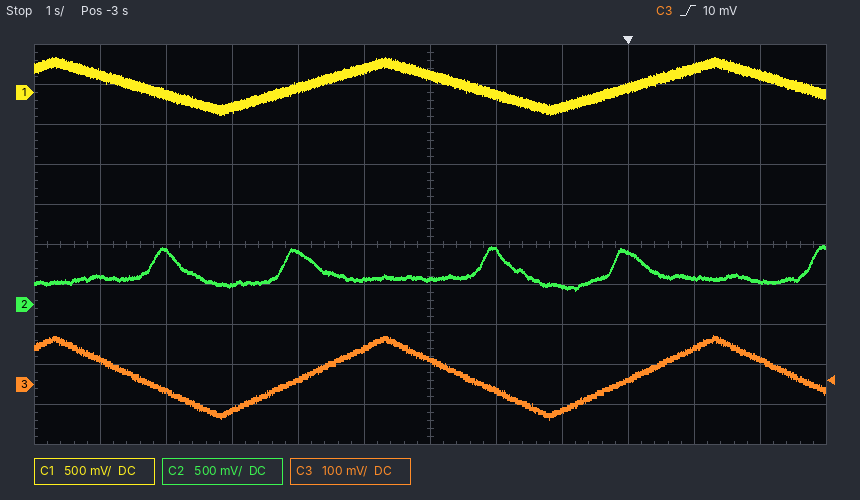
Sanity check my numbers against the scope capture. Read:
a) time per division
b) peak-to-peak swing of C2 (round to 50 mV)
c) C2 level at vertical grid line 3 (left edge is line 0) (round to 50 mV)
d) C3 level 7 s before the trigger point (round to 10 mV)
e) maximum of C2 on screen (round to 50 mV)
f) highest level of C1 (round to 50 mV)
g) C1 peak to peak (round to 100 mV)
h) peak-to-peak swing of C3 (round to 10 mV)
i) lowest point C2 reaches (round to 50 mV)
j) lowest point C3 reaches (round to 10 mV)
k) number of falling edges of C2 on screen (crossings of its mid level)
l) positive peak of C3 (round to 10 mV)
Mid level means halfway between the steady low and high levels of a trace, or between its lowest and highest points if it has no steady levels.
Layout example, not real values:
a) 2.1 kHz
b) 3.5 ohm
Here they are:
a) 1 s
b) 550 mV
c) 250 mV
d) -20 mV
e) 750 mV
f) 450 mV
g) 700 mV
h) 210 mV
i) 200 mV
j) -90 mV
k) 4
l) 120 mV
